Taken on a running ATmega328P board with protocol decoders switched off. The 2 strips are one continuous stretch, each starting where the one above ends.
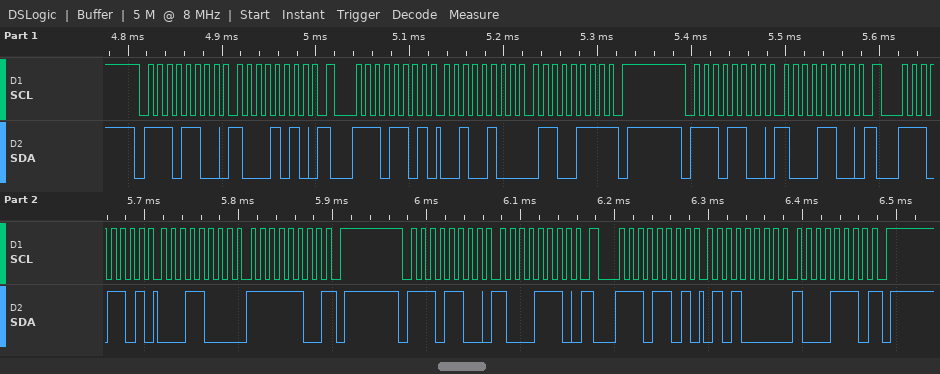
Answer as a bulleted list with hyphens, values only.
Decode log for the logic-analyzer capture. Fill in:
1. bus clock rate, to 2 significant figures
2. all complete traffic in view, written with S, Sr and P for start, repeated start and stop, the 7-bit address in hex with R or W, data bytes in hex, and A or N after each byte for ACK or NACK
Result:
- 100 kHz
- S 76W A 8A A Sr 76R A 24 A 67 N P S 76W A 8C A Sr 76R A 18 A FC N P S 76W A 8E A Sr 76R A 50 A 8E N P
